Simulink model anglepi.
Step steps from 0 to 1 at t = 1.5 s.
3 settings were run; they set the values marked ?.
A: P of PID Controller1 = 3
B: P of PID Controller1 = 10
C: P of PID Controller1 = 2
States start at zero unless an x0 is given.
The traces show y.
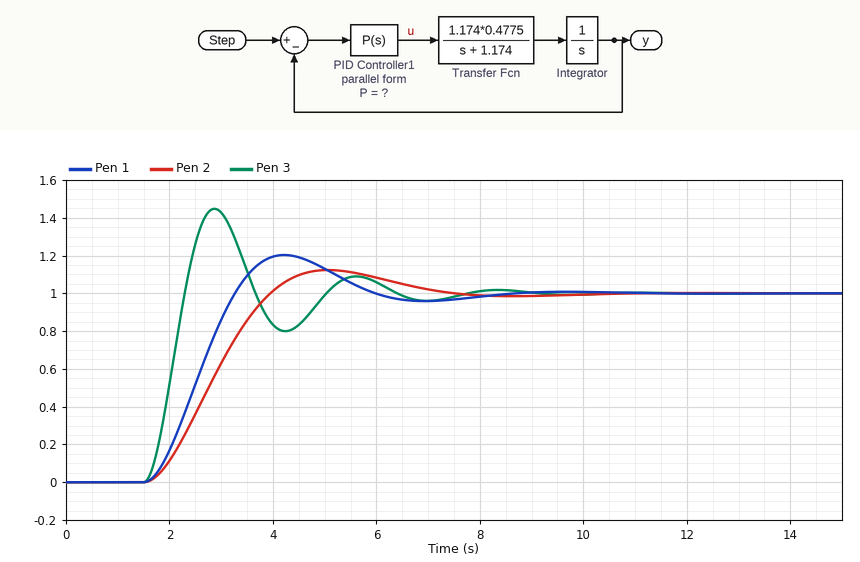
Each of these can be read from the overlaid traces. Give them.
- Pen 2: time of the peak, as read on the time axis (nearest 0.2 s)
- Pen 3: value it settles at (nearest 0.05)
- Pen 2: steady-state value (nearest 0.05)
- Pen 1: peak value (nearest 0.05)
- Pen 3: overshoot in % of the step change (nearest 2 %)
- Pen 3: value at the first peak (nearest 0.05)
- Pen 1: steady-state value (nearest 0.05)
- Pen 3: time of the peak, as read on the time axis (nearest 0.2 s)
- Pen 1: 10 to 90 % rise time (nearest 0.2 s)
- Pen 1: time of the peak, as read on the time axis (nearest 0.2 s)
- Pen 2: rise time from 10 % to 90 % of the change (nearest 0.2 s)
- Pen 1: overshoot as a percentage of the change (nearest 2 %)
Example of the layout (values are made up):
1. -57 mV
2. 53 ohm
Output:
1. 5.0 s
2. 1.00
3. 1.00
4. 1.20
5. 44 %
6. 1.45
7. 1.00
8. 2.8 s
9. 1.2 s
10. 4.2 s
11. 1.6 s
12. 20 %
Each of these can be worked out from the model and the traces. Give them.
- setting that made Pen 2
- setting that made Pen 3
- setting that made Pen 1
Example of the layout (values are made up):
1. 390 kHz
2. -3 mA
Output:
1. C
2. B
3. A
